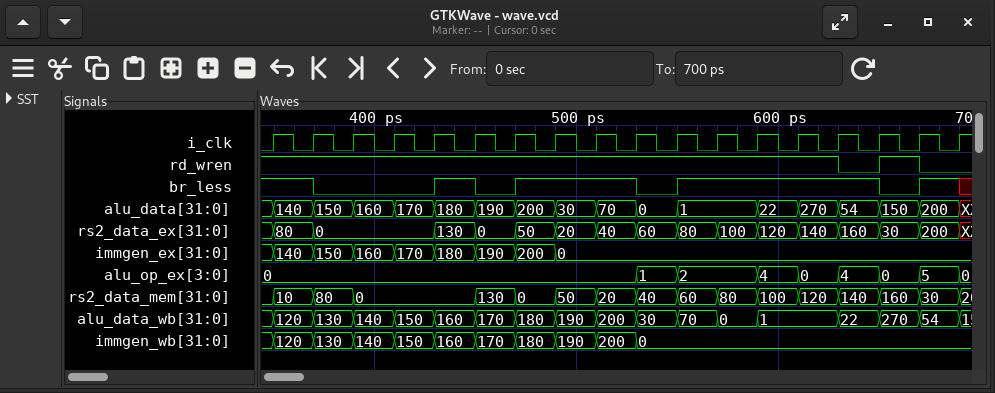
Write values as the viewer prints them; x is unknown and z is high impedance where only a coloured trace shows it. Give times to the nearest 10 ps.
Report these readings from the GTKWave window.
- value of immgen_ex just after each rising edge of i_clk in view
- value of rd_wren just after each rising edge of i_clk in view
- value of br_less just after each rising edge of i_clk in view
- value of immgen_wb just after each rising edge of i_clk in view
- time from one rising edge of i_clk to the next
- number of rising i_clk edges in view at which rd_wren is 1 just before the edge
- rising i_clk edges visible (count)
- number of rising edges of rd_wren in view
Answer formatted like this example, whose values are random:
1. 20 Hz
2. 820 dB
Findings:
1. 140, 150, 160, 170, 180, 190, 200, 0, 0, 0, 0, 0, 0, 0, 0, 0, 0, 0
2. 1 1 1 1 1 1 1 1 1 1 1 1 1 1 0 1 0 0
3. 1 0 0 0 1 0 1 1 1 0 1 1 1 1 1 0 1 x
4. 120, 130, 140, 150, 160, 170, 180, 190, 200, 0, 0, 0, 0, 0, 0, 0, 0, 0
5. 20 ps
6. 16
7. 18
8. 1
